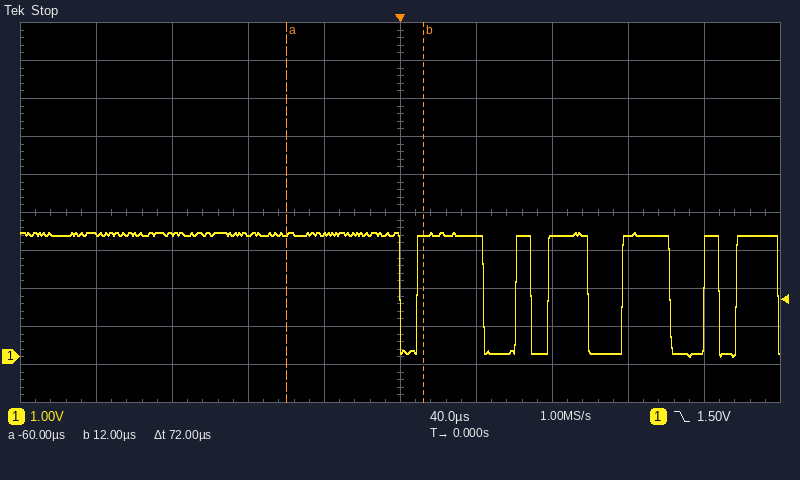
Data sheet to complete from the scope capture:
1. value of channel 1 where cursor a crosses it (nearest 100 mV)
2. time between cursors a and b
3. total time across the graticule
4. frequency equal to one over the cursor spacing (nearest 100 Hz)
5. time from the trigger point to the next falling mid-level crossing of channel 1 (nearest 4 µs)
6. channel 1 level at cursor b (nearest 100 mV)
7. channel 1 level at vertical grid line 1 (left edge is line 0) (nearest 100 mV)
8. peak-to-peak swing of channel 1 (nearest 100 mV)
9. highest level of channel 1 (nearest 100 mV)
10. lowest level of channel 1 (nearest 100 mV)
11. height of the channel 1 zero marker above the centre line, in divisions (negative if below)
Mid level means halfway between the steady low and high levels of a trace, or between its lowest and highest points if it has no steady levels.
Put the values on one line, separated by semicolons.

3.2 V; 72 µs; 400 µs; 13.9 kHz; 44 µs; 3.2 V; 3.2 V; 3.3 V; 3.3 V; 0.0 V; -3.8 div
